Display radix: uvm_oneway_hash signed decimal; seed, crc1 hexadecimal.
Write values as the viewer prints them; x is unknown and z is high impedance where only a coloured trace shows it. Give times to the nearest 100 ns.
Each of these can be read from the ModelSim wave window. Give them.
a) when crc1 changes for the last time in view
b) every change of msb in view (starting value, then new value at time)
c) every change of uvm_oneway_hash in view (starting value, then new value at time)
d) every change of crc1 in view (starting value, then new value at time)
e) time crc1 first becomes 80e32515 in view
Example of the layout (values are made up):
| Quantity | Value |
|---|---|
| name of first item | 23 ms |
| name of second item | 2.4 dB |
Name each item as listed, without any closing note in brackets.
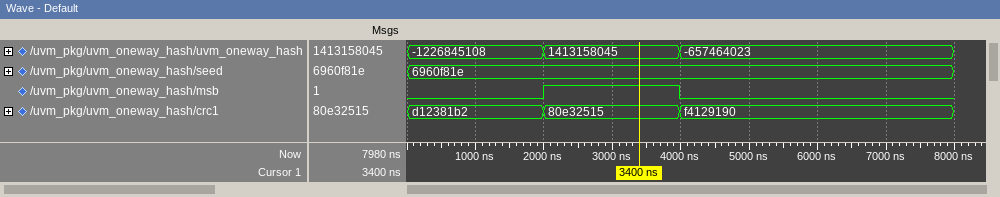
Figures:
| Quantity | Value |
|---|---|
| when crc1 changes for the last time in view | 4000 ns |
| every change of msb in view | 0, 1 at 2000 ns, 0 at 4000 ns |
| every change of uvm_oneway_hash in view | -1226845108, 1413158045 at 2000 ns, -657464023 at 4000 ns |
| every change of crc1 in view | d12381b2, 80e32515 at 2000 ns, f4129190 at 4000 ns |
| time crc1 first becomes 80e32515 in view | 2000 ns |
